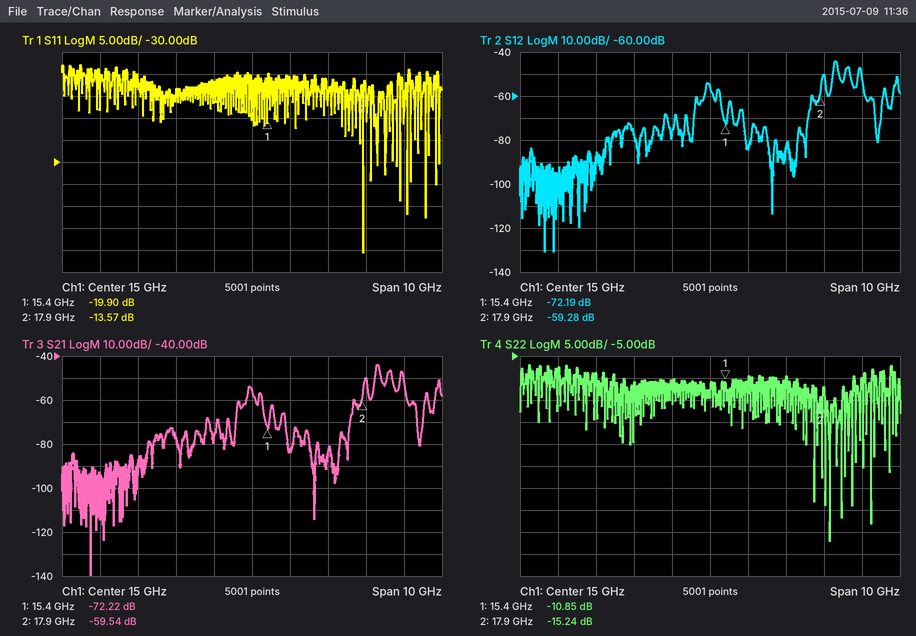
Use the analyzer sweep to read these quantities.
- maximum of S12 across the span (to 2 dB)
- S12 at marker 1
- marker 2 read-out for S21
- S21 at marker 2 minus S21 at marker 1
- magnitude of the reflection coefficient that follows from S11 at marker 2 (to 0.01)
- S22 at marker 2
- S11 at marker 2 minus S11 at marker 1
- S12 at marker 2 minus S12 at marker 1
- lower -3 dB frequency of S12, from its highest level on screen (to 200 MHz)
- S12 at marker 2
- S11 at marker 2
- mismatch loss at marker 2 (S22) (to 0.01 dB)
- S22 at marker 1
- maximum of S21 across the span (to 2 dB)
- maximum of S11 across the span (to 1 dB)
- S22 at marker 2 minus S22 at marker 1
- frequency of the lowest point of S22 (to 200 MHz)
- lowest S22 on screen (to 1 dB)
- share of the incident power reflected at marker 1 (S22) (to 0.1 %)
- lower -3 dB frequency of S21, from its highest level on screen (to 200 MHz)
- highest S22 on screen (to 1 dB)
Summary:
-44 dB
-72.19 dB
-59.54 dB
12.68 dB
0.21
-15.24 dB
6.33 dB
12.91 dB
18.2 GHz
-59.28 dB
-13.57 dB
0.13 dB
-10.85 dB
-44 dB
-8 dB
-4.39 dB
18.2 GHz
-47 dB
8.2 %
18.2 GHz
-7 dB
